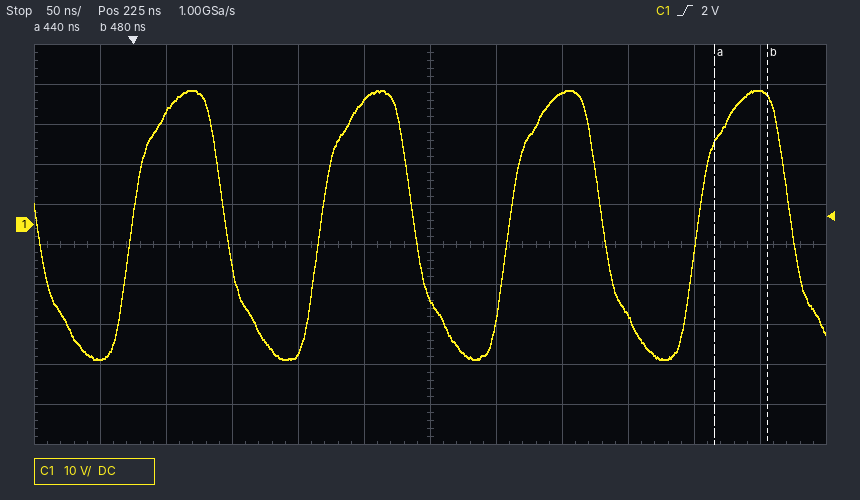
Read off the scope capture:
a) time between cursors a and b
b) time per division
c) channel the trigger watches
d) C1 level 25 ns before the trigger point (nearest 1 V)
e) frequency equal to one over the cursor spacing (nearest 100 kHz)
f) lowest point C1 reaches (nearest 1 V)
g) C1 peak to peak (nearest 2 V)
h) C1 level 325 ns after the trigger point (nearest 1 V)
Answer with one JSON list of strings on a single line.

["40 ns", "50 ns", "C1", "-34 V", "25.0 MHz", "-34 V", "68 V", "33 V"]
